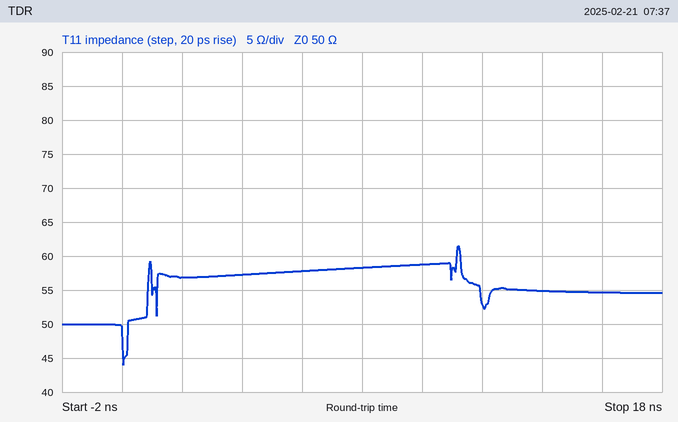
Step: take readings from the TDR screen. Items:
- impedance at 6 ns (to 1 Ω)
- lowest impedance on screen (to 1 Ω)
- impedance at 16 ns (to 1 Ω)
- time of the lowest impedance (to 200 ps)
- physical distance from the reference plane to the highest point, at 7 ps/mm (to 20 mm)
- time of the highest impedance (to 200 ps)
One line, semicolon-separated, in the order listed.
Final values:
58 Ω; 44 Ω; 55 Ω; 0.0 ns; 800 mm; 11.2 ns
